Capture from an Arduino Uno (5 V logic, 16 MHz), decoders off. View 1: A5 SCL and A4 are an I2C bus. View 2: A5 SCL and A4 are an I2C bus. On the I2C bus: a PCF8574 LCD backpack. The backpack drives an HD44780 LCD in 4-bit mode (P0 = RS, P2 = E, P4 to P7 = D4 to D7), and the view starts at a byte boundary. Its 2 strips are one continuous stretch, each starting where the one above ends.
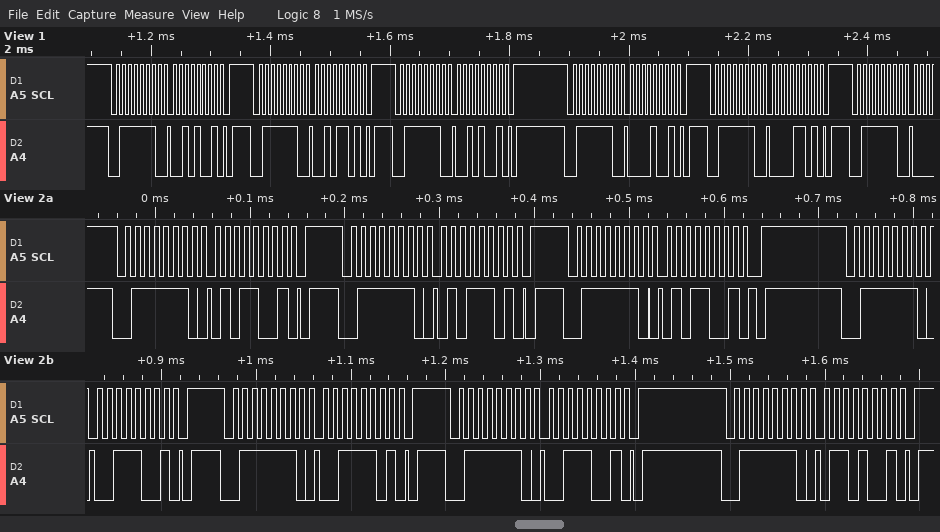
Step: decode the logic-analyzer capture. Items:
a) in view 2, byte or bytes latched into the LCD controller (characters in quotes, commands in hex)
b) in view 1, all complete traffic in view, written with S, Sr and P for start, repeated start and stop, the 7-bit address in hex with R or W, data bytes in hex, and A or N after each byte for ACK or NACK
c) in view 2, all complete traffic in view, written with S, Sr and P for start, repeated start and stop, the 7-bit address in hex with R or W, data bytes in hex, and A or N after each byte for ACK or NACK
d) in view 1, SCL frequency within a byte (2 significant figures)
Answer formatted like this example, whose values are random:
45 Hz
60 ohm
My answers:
'S'
S 3FW A 29 A P S 3FW A 2D A P S 3FW A 29 A P S 3FW A 09 A P S 3FW A 0D A P S 3FW A
S 3FW A 59 A P S 3FW A 5D A P S 3FW A 59 A P S 3FW A 39 A P S 3FW A 3D A P S 3FW A 39 A P S 3FW A 69 A P
100 kHz
